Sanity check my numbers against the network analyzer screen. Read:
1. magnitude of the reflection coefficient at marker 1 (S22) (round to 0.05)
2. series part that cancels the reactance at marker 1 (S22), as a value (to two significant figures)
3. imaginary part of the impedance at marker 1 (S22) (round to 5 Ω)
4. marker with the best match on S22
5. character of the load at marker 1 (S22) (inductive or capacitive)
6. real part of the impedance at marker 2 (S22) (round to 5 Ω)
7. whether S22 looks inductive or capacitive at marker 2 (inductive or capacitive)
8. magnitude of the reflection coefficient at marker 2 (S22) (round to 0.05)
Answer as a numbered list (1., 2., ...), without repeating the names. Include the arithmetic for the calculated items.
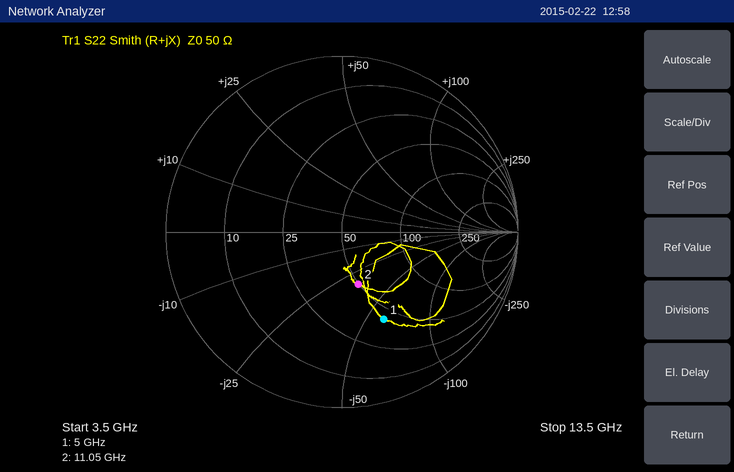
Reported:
1. 0.55
2. L = 60 Ω/(2π × 5 GHz) ≈ 1.9 nH
3. -60 Ω
4. marker 2
5. capacitive
6. 50 Ω
7. capacitive
8. 0.30
